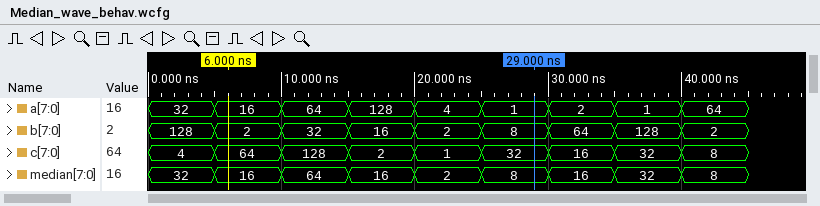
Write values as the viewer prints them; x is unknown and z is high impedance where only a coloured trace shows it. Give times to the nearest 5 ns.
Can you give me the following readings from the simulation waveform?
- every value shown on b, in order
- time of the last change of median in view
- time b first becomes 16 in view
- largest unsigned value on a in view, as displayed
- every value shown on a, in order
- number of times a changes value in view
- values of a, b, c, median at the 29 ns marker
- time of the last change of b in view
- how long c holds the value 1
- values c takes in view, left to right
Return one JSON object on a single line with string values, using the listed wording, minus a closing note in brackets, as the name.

{"every value shown on b, in order": "128, 2, 32, 16, 2, 8, 64, 128, 2", "time of the last change of median in view": "40 ns", "time b first becomes 16 in view": "15 ns", "largest unsigned value on a in view, as displayed": "128", "every value shown on a, in order": "32, 16, 64, 128, 4, 1, 2, 1, 64", "number of times a changes value in view": "8", "values of a, b, c, median at the 29 ns marker": "a=1, b=8, c=32, median=8", "time of the last change of b in view": "40 ns", "how long c holds the value 1": "5 ns", "values c takes in view, left to right": "4, 64, 128, 2, 1, 32, 16, 32, 8"}
